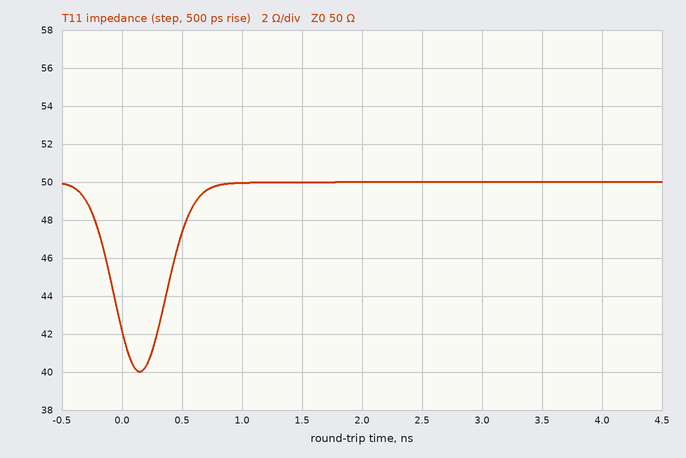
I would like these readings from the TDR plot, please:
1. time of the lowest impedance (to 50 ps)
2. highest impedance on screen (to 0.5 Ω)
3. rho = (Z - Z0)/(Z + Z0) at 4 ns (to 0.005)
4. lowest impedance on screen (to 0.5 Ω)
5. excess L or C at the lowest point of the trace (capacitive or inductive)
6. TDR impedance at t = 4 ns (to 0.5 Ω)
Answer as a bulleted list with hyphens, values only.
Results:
- 150 ps
- 50.0 Ω
- 0.000
- 40.0 Ω
- capacitive
- 50.0 Ω
